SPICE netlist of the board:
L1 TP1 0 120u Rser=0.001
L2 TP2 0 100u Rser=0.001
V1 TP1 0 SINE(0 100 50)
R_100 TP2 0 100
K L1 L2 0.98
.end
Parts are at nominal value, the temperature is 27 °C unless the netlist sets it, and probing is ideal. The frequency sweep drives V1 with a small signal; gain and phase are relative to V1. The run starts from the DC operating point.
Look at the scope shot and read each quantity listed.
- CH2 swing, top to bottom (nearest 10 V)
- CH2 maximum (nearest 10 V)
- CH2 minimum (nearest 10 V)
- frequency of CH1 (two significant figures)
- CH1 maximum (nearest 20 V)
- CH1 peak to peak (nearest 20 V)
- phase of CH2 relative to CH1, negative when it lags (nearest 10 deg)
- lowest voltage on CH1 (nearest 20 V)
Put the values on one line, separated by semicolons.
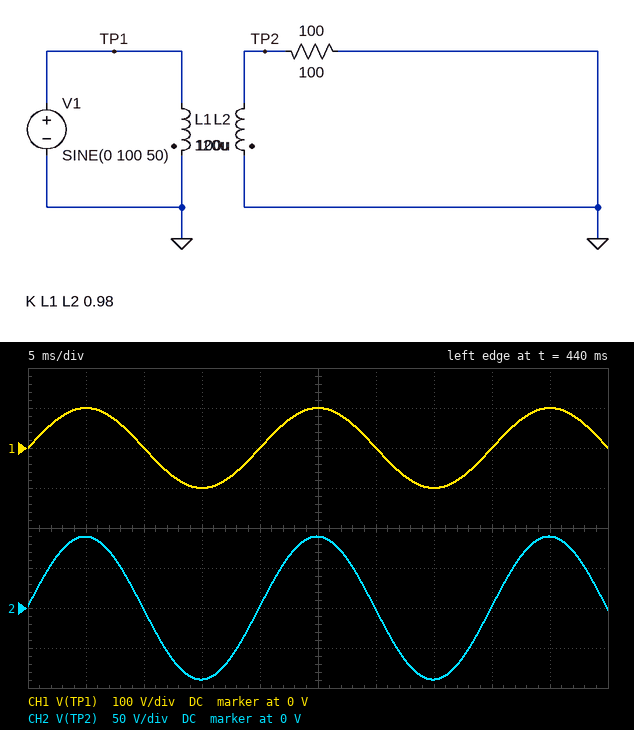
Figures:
180 V; 90 V; -90 V; 50 Hz; 100 V; 200 V; 0 deg; -100 V
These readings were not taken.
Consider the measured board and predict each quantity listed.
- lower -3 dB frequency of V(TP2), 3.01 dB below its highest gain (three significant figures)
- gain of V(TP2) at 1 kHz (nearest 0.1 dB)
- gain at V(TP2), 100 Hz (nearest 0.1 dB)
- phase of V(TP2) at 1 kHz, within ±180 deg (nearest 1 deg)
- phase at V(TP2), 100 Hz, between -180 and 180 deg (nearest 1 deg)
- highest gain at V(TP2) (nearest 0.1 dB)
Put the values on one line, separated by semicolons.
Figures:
1.33 Hz; -1.0 dB; -1.0 dB; 0 deg; 1 deg; -1.0 dB
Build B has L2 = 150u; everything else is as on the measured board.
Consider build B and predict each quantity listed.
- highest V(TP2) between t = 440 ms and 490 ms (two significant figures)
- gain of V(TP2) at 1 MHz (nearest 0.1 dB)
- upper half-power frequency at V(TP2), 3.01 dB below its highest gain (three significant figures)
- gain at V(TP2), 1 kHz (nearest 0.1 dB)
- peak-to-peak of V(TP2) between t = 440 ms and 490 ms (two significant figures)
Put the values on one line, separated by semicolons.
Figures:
110 V; 0.2 dB; 2.68 MHz; 0.8 dB; 220 V
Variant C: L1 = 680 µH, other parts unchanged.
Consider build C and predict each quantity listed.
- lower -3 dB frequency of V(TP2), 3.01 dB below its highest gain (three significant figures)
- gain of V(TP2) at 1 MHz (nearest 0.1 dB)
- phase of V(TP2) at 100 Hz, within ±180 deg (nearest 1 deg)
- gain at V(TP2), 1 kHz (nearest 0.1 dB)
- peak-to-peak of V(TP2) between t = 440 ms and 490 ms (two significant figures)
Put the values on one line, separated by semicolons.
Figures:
234 mHz; -8.8 dB; 0 deg; -8.5 dB; 75 V
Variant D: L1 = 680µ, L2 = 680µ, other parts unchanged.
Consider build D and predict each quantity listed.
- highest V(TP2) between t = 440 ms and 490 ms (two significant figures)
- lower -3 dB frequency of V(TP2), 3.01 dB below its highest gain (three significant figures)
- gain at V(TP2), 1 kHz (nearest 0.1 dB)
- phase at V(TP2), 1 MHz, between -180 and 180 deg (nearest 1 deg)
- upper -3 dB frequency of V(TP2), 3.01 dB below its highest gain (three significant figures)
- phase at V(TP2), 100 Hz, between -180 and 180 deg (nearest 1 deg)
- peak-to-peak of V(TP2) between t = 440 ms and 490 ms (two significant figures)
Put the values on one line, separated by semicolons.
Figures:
98 V; 234 mHz; -0.2 dB; -59 deg; 591 kHz; 0 deg; 200 V
